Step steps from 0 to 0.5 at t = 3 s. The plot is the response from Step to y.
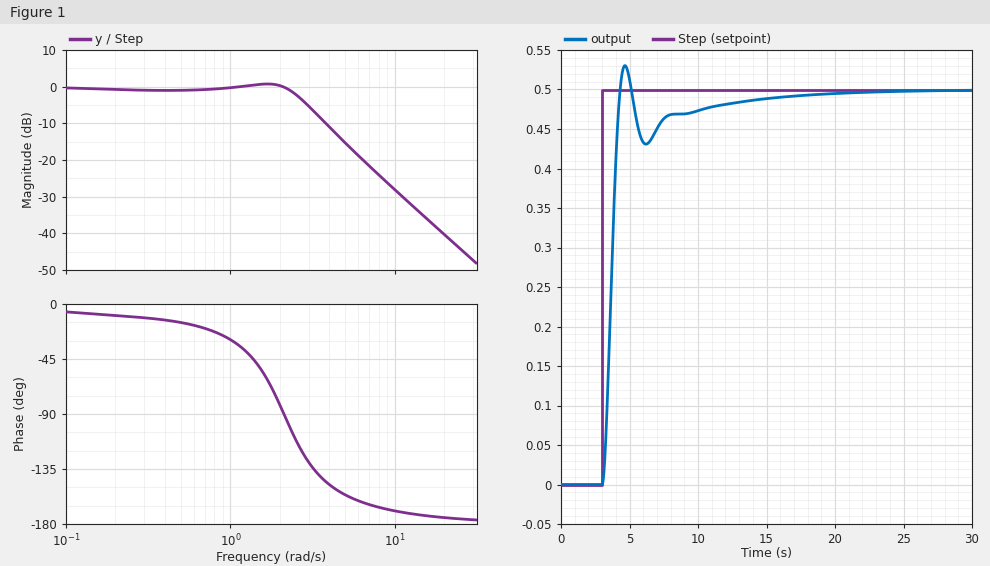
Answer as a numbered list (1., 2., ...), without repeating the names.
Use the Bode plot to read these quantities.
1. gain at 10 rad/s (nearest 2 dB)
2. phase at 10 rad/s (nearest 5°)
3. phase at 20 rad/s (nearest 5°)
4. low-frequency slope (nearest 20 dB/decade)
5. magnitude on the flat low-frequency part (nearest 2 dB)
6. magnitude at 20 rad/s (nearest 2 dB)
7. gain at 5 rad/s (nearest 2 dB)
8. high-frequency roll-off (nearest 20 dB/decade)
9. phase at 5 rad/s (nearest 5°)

1. -28 dB
2. -170°
3. -175°
4. 0 dB/decade
5. 0 dB
6. -40 dB
7. -16 dB
8. -40 dB/decade
9. -155°
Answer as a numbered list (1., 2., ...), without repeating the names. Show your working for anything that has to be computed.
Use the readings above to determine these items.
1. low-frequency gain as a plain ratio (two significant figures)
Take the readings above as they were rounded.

1. 10^(0 / 20) = 1.0
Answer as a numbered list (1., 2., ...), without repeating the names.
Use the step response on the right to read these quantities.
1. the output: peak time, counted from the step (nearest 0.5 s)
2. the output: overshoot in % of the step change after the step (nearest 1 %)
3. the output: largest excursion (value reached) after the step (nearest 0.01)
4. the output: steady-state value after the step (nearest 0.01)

1. 1.5 s
2. 6 %
3. 0.53
4. 0.50
